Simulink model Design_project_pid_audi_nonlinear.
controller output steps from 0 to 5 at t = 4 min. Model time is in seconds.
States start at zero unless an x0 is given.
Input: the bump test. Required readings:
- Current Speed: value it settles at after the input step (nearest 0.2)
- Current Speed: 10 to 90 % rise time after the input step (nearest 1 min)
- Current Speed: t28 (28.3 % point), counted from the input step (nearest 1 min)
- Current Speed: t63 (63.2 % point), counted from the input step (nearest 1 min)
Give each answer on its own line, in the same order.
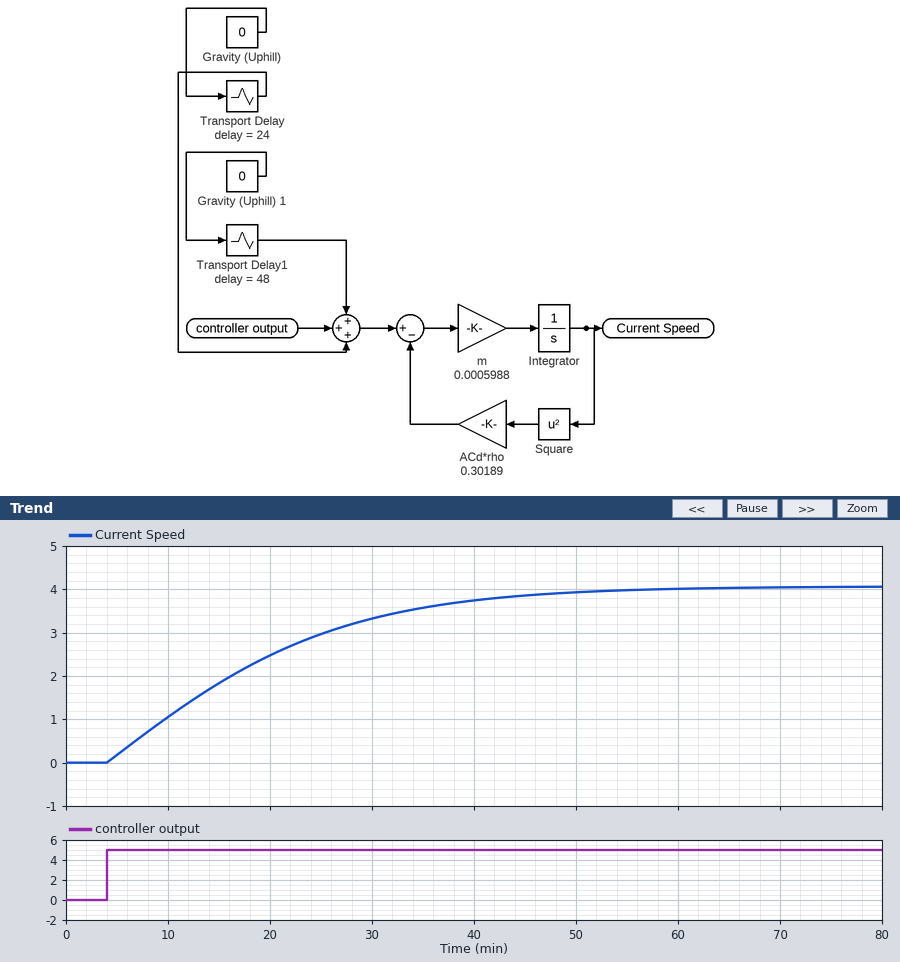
4.0
31 min
7 min
17 min
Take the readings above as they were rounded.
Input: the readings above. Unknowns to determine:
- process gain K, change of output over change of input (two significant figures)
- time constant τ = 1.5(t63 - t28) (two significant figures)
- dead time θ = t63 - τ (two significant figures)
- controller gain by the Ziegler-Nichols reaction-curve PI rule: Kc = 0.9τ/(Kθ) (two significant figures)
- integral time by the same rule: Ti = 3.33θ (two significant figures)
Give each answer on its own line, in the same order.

0.80
15 min
2.0 min
8.4
6.7 min
